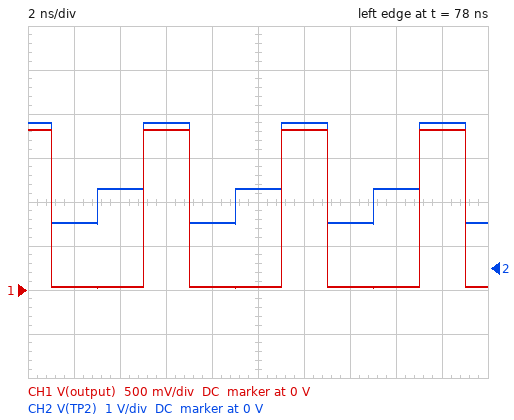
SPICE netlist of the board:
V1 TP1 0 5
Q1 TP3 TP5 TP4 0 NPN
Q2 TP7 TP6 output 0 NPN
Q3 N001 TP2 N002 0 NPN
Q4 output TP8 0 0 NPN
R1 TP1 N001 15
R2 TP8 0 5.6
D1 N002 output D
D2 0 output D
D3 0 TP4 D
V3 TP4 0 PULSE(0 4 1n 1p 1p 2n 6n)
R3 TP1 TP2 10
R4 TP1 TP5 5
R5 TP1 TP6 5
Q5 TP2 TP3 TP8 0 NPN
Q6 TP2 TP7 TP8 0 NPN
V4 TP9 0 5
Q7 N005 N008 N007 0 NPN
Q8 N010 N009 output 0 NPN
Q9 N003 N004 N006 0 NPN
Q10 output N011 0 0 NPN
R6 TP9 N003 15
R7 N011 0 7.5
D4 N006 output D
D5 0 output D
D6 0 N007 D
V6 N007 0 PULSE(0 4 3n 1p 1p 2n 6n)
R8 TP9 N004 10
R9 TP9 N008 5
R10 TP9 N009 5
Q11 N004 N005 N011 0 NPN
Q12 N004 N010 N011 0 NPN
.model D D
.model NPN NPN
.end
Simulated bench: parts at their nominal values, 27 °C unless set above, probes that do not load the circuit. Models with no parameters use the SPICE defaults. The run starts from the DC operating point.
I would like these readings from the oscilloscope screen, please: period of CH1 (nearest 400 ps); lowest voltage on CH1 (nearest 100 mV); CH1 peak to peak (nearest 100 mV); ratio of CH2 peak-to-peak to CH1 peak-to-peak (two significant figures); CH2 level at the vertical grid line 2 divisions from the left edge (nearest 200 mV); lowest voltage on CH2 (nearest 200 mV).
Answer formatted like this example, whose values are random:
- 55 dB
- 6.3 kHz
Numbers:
- 6.0 ns
- 0 V
- 1.8 V
- 1.3
- 1.8 V
- 1.0 V
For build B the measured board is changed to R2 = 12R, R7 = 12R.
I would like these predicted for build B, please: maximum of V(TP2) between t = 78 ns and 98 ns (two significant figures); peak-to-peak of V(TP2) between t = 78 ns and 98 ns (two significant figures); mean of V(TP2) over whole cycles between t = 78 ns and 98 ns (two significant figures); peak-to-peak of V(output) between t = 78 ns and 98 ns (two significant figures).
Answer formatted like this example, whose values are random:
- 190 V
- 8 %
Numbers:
- 3.5 V
- 2.5 V
- 2.1 V
- 1.8 V
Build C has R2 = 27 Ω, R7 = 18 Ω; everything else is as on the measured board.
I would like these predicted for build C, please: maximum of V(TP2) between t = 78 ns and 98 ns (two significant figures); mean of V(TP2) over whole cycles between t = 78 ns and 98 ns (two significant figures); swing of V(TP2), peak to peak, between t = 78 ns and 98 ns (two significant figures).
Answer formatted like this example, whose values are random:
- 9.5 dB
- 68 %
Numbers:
- 3.5 V
- 2.1 V
- 2.5 V
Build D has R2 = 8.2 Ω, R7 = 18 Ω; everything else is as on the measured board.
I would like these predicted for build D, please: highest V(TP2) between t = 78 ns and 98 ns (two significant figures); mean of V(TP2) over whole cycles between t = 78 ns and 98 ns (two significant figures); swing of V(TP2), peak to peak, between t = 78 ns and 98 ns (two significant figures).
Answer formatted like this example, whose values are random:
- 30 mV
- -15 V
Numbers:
- 3.5 V
- 2.1 V
- 2.5 V
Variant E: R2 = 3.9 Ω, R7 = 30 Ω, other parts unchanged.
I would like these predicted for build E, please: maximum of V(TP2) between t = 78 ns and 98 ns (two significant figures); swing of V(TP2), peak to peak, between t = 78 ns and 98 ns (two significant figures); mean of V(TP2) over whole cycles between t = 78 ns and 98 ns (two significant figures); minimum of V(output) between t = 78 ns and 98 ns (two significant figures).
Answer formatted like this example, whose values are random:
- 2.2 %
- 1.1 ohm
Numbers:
- 2.7 V
- 1.7 V
- 1.8 V
- 26 mV
